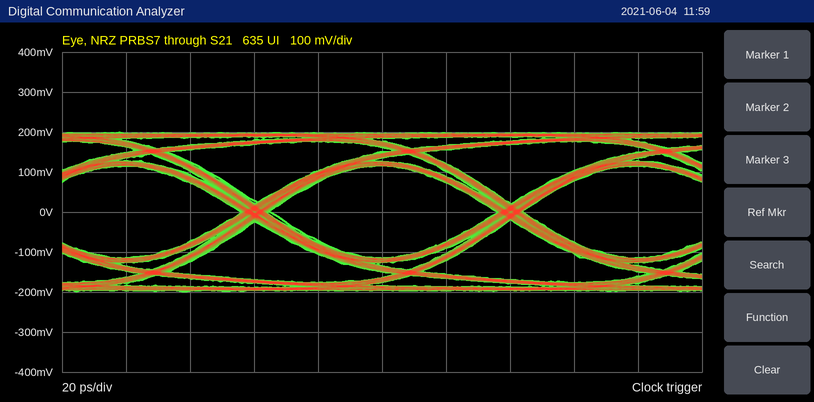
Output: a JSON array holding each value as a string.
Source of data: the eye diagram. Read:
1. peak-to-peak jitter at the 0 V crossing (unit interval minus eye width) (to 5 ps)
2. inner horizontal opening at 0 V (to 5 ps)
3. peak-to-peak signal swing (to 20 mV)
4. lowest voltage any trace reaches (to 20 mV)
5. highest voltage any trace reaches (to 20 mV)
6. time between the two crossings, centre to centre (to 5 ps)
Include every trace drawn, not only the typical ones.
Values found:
["10 ps", "70 ps", "400 mV", "-200 mV", "200 mV", "80 ps"]
